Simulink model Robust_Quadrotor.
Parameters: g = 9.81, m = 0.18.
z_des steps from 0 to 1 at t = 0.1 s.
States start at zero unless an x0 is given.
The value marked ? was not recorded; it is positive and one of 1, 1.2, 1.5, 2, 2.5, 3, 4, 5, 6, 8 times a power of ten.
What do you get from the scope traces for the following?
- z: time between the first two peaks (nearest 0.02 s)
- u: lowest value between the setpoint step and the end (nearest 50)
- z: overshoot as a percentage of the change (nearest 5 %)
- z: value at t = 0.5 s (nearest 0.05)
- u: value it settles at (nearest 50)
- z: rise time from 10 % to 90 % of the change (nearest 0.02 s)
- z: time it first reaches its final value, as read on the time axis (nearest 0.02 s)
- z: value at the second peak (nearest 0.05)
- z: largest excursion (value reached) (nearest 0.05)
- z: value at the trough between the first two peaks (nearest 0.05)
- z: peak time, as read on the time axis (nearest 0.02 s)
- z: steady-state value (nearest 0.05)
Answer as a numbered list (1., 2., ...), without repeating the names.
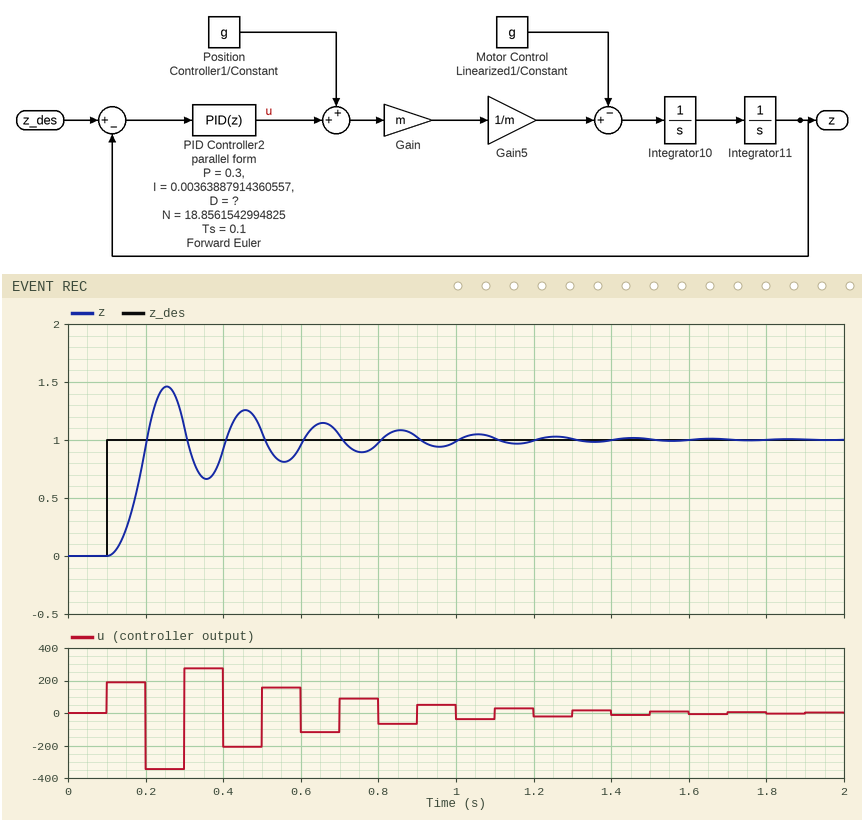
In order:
1. 0.20 s
2. -350
3. 45 %
4. 1.05
5. 0
6. 0.06 s
7. 0.20 s
8. 1.25
9. 1.45
10. 0.65
11. 0.26 s
12. 1.00
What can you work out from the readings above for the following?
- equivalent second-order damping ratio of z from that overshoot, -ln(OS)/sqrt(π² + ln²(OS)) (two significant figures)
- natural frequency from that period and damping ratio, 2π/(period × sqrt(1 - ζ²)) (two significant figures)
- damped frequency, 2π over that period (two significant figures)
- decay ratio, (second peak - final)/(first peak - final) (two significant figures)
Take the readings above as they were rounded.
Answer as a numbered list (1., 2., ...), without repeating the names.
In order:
1. 0.25
2. 32 rad/s
3. 31 rad/s
4. 0.56
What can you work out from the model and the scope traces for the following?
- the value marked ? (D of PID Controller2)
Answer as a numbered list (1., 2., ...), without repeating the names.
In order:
1. 10
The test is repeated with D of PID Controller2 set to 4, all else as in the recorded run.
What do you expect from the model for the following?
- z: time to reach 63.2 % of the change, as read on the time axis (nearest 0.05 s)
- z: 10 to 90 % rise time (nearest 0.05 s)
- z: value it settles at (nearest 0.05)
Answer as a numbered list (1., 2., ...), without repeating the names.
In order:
1. 0.25 s
2. 0.30 s
3. 1.00
